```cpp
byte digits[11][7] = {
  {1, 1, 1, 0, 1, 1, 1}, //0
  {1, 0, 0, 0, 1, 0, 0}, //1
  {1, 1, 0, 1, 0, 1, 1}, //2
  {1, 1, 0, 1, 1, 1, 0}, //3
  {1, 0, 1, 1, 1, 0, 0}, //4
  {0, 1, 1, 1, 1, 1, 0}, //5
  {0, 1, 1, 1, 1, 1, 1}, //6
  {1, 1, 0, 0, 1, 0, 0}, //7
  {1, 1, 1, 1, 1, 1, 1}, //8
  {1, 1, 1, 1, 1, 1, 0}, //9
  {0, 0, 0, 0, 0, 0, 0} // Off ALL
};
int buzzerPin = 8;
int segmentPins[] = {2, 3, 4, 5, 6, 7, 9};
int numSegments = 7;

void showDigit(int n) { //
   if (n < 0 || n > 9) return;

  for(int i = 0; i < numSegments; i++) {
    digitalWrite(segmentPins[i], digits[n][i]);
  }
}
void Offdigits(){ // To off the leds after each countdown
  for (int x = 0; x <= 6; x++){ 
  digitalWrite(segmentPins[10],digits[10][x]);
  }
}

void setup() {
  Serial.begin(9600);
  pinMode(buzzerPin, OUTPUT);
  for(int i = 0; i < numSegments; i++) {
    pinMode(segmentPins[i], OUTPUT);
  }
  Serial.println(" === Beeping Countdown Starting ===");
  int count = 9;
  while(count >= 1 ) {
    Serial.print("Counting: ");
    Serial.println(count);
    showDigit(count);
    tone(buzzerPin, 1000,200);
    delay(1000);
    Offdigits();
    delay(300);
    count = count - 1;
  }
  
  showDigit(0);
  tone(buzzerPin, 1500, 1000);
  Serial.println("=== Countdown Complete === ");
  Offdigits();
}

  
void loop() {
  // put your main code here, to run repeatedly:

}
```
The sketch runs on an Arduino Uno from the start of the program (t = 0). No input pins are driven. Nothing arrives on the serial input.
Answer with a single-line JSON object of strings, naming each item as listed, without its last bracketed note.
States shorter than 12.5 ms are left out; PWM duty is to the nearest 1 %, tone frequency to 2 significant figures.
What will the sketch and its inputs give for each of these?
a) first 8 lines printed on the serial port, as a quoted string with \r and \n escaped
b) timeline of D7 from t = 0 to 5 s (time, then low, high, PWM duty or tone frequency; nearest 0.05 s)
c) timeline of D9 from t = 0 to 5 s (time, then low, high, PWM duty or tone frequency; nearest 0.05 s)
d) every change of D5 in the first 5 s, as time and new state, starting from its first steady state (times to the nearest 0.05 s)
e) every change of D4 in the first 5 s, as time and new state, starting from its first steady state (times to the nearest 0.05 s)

{"first 8 lines printed on the serial port, as a quoted string with \\r and \\n escaped": "\" === Beeping Countdown Starting ===\\r\\nCounting: 9\\r\\nCounting: 8\\r\\nCounting: 7\\r\\nCounting: 6\\r\\nCounting: 5\\r\\nCounting: 4\\r\\nCounting: 3\\r\\n\"", "timeline of D7 from t = 0 to 5 s": "0 s high; 2.6 s low; 3.9 s high", "timeline of D9 from t = 0 to 5 s": "0 s low; 1.3 s high; 2.6 s low; 3.9 s high", "every change of D5 in the first 5 s, as time and new state, starting from its first steady state": "0 s high; 2.6 s low; 3.9 s high", "every change of D4 in the first 5 s, as time and new state, starting from its first steady state": "0 s high; 2.6 s low; 3.9 s high"}
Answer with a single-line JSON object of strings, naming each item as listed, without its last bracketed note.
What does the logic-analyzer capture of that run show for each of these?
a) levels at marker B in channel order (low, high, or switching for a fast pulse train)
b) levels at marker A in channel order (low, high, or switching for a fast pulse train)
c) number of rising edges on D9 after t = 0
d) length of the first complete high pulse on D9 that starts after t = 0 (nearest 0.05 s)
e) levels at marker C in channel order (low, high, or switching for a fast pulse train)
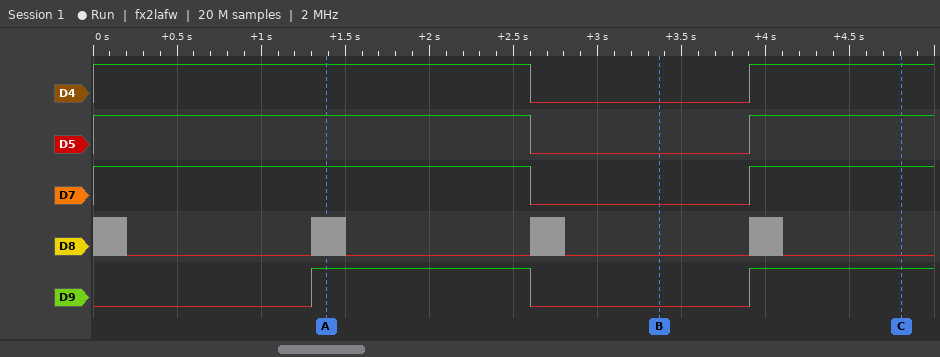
{"levels at marker B in channel order": "D4 low, D5 low, D7 low, D8 low, D9 low", "levels at marker A in channel order": "D4 high, D5 high, D7 high, D8 switching, D9 high", "number of rising edges on D9 after t = 0": "2", "length of the first complete high pulse on D9 that starts after t = 0": "1.30 s", "levels at marker C in channel order": "D4 high, D5 high, D7 high, D8 low, D9 high"}
